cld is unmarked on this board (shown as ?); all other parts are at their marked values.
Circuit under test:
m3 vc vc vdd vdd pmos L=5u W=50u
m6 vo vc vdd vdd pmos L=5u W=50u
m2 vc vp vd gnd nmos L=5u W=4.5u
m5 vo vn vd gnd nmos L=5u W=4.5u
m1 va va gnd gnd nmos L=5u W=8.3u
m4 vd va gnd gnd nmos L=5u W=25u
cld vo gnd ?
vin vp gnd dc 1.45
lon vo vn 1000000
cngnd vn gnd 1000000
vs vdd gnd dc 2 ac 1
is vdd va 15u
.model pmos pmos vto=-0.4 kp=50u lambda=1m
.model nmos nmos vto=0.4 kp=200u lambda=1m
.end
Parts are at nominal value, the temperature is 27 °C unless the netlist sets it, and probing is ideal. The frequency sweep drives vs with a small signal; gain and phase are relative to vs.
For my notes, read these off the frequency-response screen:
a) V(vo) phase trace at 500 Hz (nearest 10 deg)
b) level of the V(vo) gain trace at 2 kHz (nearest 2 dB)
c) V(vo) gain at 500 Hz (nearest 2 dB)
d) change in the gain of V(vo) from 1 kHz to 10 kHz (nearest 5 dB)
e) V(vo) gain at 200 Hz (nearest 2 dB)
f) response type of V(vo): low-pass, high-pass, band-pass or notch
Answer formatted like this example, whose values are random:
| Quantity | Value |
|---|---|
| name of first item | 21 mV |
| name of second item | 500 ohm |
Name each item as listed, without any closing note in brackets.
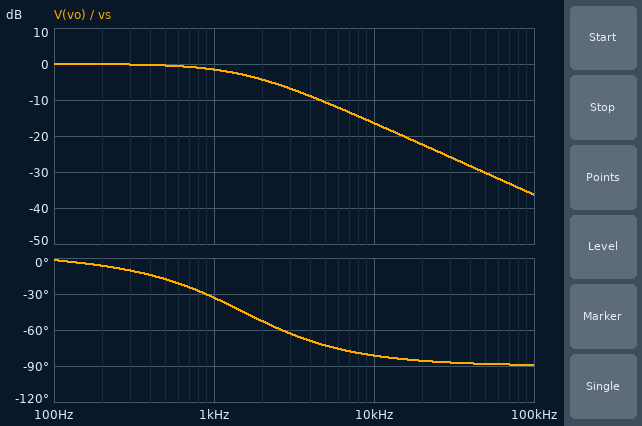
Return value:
| Quantity | Value |
|---|---|
| V(vo) phase trace at 500 Hz | -20 deg |
| level of the V(vo) gain trace at 2 kHz | -4 dB |
| V(vo) gain at 500 Hz | 0 dB |
| change in the gain of V(vo) from 1 kHz to 10 kHz | -15 dB |
| V(vo) gain at 200 Hz | 0 dB |
| response type of V(vo): low-pass, high-pass, band-pass or notch | low-pass |
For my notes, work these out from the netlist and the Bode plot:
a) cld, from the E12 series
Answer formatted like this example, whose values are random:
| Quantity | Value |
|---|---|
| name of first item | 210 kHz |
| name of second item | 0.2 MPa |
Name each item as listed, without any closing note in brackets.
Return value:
| Quantity | Value |
|---|---|
| cld, from the E12 series | 4.7 pF |
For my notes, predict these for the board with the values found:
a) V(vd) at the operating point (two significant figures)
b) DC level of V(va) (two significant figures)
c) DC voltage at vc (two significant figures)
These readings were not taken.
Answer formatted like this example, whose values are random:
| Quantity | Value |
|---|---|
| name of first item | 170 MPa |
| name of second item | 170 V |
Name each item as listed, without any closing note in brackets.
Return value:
| Quantity | Value |
|---|---|
| V(vd) at the operating point | 550 mV |
| DC level of V(va) | 700 mV |
| DC voltage at vc | 1.3 V |
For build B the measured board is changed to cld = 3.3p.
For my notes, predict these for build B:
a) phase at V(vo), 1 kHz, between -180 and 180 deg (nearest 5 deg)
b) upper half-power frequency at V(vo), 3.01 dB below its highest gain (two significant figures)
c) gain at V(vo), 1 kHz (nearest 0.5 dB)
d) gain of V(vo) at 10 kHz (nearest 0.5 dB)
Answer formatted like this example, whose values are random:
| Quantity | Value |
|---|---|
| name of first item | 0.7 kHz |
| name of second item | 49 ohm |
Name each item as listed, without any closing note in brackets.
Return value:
| Quantity | Value |
|---|---|
| phase at V(vo), 1 kHz, between -180 and 180 deg | -25 deg |
| upper half-power frequency at V(vo), 3.01 dB below its highest gain | 2.2 kHz |
| gain at V(vo), 1 kHz | -1.0 dB |
| gain of V(vo) at 10 kHz | -13.5 dB |
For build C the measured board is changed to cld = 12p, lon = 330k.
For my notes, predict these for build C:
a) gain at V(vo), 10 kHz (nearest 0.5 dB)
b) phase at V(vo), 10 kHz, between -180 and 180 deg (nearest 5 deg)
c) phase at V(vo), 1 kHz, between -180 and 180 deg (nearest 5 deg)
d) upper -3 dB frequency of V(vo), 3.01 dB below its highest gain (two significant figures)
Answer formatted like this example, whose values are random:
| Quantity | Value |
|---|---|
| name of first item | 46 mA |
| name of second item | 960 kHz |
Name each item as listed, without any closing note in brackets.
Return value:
| Quantity | Value |
|---|---|
| gain at V(vo), 10 kHz | -24.5 dB |
| phase at V(vo), 10 kHz, between -180 and 180 deg | -85 deg |
| phase at V(vo), 1 kHz, between -180 and 180 deg | -60 deg |
| upper -3 dB frequency of V(vo), 3.01 dB below its highest gain | 610 Hz |
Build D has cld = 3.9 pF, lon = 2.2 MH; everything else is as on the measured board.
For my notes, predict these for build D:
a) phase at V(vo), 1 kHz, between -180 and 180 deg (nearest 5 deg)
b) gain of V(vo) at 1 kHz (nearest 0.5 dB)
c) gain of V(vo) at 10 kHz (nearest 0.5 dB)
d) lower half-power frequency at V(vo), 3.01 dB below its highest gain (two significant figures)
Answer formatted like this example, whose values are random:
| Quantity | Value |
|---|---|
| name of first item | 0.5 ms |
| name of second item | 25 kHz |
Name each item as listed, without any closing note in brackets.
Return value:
| Quantity | Value |
|---|---|
| phase at V(vo), 1 kHz, between -180 and 180 deg | -30 deg |
| gain of V(vo) at 1 kHz | -1.0 dB |
| gain of V(vo) at 10 kHz | -15.0 dB |
| lower half-power frequency at V(vo), 3.01 dB below its highest gain | 1.6 Hz |
